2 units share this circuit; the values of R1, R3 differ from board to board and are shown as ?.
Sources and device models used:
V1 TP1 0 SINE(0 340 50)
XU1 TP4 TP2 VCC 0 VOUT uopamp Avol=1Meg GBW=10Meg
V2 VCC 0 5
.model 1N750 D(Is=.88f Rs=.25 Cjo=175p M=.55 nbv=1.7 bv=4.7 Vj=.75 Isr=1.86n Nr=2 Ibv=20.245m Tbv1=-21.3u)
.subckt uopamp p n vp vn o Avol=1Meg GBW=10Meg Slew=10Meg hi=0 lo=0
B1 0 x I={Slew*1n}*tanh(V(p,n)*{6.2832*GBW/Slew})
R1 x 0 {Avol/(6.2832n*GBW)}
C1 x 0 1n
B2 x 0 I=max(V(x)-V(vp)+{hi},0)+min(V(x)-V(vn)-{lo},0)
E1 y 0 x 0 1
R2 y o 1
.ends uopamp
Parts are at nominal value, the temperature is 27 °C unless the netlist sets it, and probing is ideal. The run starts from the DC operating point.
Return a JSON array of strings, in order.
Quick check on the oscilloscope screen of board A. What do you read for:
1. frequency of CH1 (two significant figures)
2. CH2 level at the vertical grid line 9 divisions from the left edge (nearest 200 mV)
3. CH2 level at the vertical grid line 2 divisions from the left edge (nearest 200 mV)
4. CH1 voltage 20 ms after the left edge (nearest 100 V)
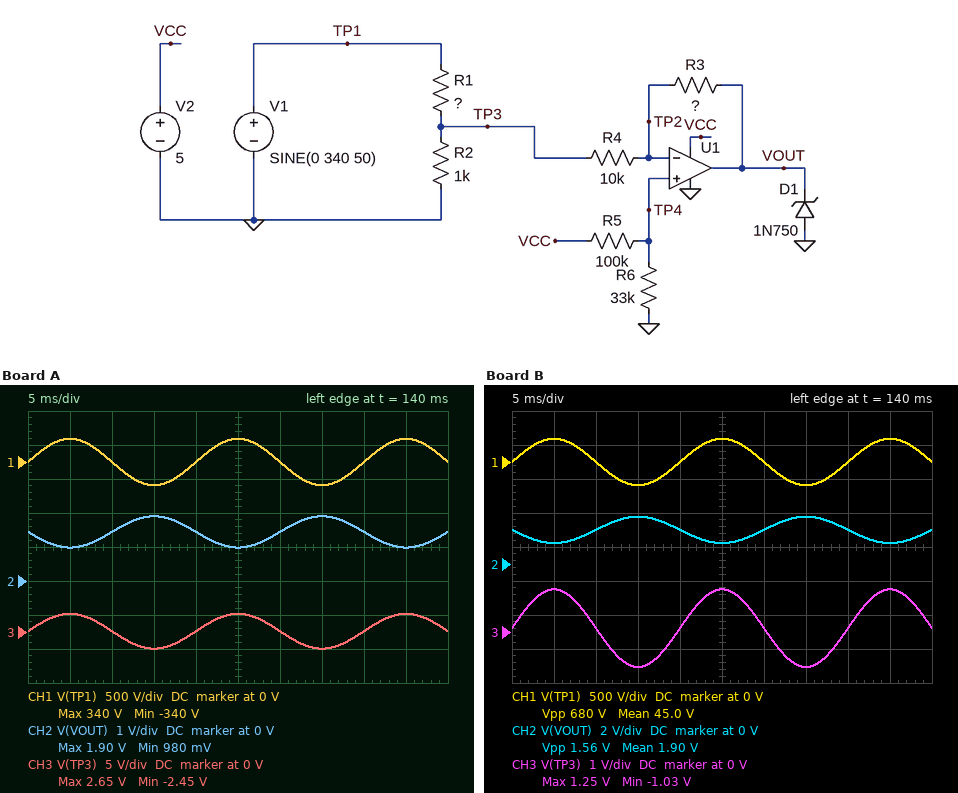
["50 Hz", "1.0 V", "1.4 V", "0 V"]
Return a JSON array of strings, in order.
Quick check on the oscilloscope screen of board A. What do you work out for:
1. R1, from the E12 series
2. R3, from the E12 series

["120 kΩ", "1.8 kΩ"]
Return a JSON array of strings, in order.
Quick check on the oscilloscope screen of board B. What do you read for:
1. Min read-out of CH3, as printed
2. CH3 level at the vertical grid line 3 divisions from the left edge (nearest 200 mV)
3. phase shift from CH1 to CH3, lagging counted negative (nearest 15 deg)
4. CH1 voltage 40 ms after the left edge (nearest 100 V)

["-1.03 V", "-1.0 V", "0 deg", "0 V"]
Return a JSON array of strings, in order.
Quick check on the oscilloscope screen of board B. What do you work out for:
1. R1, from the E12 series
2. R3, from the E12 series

["270 kΩ", "6.8 kΩ"]
